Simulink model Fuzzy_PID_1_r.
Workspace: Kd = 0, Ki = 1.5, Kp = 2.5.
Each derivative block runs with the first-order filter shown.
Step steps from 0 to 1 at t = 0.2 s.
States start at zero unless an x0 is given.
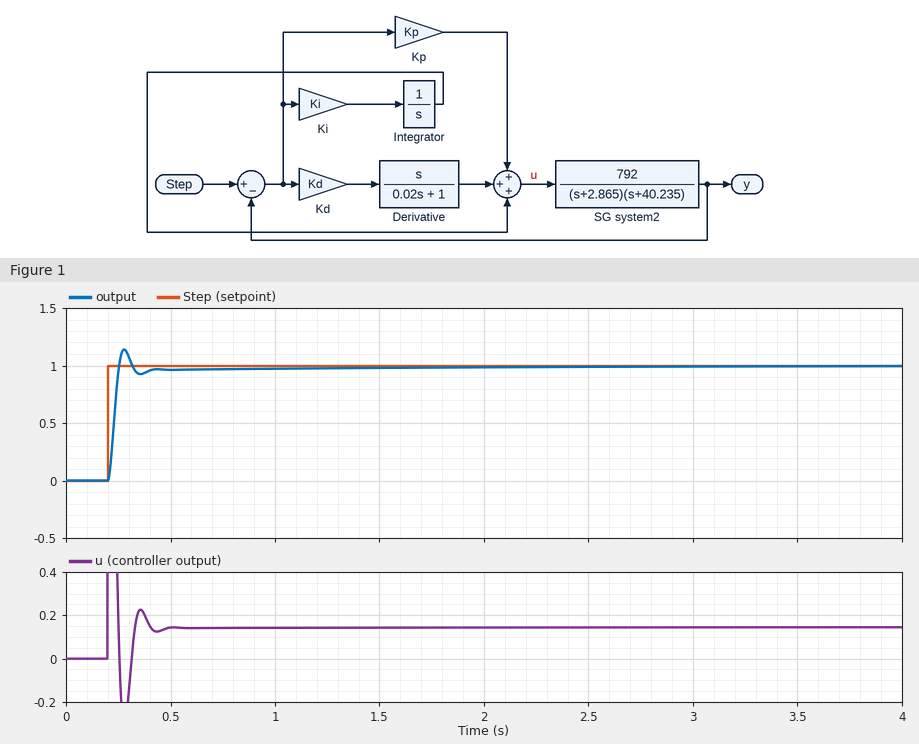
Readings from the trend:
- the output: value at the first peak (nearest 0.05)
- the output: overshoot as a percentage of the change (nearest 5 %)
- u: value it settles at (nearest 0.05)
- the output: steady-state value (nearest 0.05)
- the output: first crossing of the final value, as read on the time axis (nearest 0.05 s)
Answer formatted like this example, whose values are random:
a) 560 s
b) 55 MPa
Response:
a) 1.15
b) 15 %
c) 0.15
d) 1.00
e) 0.25 s
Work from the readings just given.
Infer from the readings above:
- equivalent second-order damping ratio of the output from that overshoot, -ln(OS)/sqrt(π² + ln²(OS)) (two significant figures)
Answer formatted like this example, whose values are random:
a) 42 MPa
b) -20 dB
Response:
a) 0.52
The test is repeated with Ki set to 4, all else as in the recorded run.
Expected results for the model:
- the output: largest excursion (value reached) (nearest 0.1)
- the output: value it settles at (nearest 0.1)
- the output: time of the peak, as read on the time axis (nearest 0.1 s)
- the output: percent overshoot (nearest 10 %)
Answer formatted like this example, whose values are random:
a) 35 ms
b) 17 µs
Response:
a) 1.2
b) 1.0
c) 0.3 s
d) 20 %
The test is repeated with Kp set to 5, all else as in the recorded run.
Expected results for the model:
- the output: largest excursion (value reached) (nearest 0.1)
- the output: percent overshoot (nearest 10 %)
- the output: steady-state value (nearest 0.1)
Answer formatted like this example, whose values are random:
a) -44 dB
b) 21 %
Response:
a) 1.3
b) 30 %
c) 1.0
